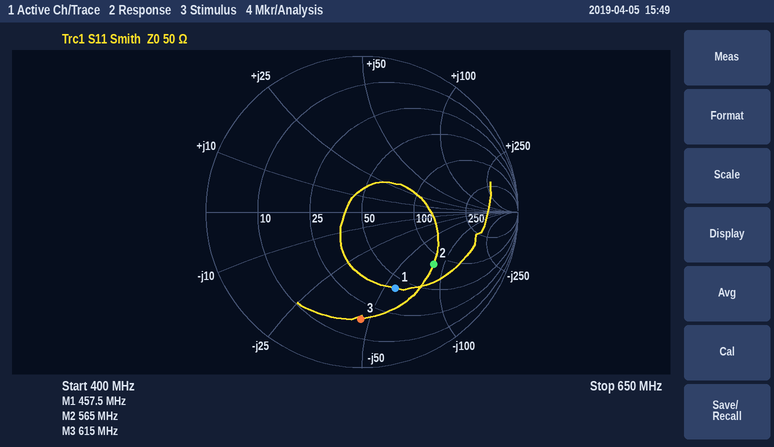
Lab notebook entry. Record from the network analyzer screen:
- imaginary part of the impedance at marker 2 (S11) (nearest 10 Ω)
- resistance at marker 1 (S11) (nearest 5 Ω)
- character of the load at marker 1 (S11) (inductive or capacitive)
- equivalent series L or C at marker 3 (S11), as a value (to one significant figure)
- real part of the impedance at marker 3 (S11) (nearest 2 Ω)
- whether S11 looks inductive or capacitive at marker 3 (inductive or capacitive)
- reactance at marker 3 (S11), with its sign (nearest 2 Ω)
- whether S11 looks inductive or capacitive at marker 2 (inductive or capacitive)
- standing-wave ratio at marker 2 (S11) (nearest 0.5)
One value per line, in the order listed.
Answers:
-80 Ω
40 Ω
capacitive
6 pF
18 Ω
capacitive
-46 Ω
capacitive
3.5
